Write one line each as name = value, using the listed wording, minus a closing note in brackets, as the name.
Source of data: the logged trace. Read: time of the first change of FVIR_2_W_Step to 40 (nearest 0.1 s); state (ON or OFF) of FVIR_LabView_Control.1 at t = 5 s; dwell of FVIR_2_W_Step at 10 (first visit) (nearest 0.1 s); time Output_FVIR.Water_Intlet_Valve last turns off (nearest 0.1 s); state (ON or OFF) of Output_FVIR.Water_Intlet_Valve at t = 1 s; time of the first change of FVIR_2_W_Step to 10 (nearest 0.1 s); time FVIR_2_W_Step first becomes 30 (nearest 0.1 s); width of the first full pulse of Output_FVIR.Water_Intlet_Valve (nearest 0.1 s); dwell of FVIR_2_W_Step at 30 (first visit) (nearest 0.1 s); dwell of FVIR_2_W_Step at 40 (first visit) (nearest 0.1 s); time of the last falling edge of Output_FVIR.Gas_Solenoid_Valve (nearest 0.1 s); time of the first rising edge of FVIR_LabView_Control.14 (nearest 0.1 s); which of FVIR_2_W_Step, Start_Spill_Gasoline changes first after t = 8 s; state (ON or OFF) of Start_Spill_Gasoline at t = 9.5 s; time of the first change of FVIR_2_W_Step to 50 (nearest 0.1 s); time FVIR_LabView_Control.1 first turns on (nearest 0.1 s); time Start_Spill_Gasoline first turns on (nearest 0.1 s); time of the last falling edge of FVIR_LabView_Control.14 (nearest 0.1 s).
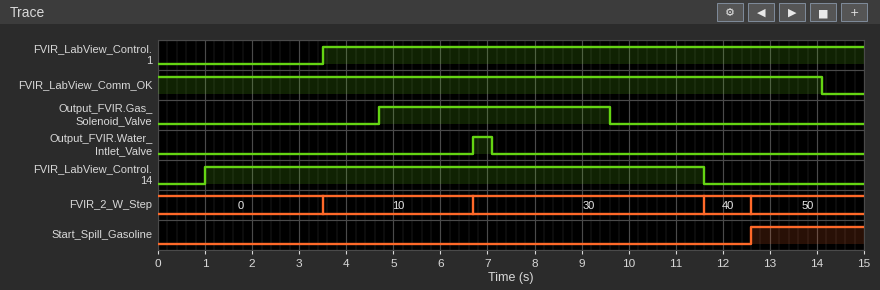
time of the first change of FVIR_2_W_Step to 40 = 11.6 s
state (ON or OFF) of FVIR_LabView_Control.1 at t = 5 s = ON
dwell of FVIR_2_W_Step at 10 (first visit) = 3.2 s
time Output_FVIR.Water_Intlet_Valve last turns off = 7.1 s
state (ON or OFF) of Output_FVIR.Water_Intlet_Valve at t = 1 s = OFF
time of the first change of FVIR_2_W_Step to 10 = 3.5 s
time FVIR_2_W_Step first becomes 30 = 6.7 s
width of the first full pulse of Output_FVIR.Water_Intlet_Valve = 0.4 s
dwell of FVIR_2_W_Step at 30 (first visit) = 4.9 s
dwell of FVIR_2_W_Step at 40 (first visit) = 1.0 s
time of the last falling edge of Output_FVIR.Gas_Solenoid_Valve = 9.6 s
time of the first rising edge of FVIR_LabView_Control.14 = 1.0 s
which of FVIR_2_W_Step, Start_Spill_Gasoline changes first after t = 8 s = FVIR_2_W_Step
state (ON or OFF) of Start_Spill_Gasoline at t = 9.5 s = OFF
time of the first change of FVIR_2_W_Step to 50 = 12.6 s
time FVIR_LabView_Control.1 first turns on = 3.5 s
time Start_Spill_Gasoline first turns on = 12.6 s
time of the last falling edge of FVIR_LabView_Control.14 = 11.6 s
